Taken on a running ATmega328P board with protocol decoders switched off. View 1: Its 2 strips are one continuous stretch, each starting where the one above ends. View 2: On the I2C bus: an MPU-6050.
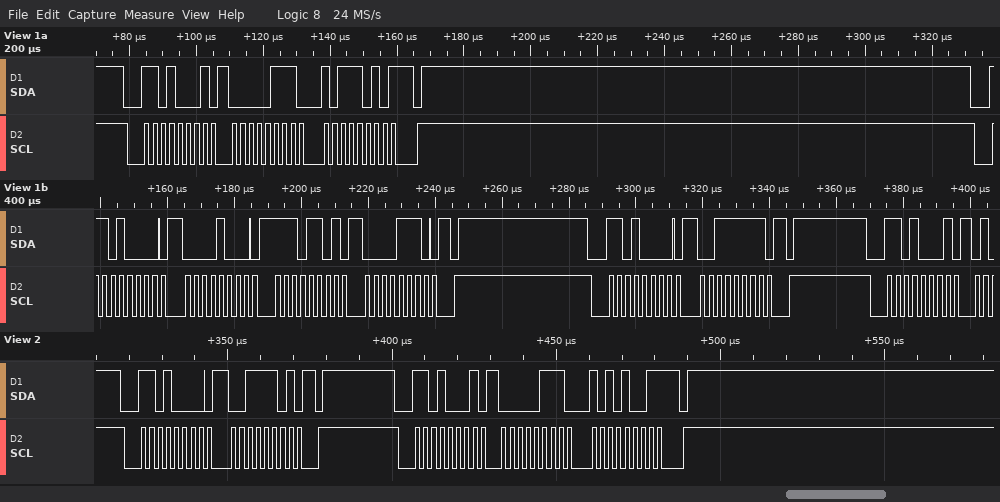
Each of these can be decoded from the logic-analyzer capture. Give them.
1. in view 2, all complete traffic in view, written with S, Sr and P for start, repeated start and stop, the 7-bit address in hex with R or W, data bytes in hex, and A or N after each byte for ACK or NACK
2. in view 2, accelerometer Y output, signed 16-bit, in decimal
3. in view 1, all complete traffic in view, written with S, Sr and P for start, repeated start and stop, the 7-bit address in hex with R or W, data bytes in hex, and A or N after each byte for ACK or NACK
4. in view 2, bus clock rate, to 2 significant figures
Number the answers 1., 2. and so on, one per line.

1. S 68W A 3D A P S 68R A 07 A A9 N P
2. 1961
3. S 68R A 07 A BA N P S 68W A 08 A ED A 0E A P S 68W A 3F A P S 68R A
4. 400 kHz
